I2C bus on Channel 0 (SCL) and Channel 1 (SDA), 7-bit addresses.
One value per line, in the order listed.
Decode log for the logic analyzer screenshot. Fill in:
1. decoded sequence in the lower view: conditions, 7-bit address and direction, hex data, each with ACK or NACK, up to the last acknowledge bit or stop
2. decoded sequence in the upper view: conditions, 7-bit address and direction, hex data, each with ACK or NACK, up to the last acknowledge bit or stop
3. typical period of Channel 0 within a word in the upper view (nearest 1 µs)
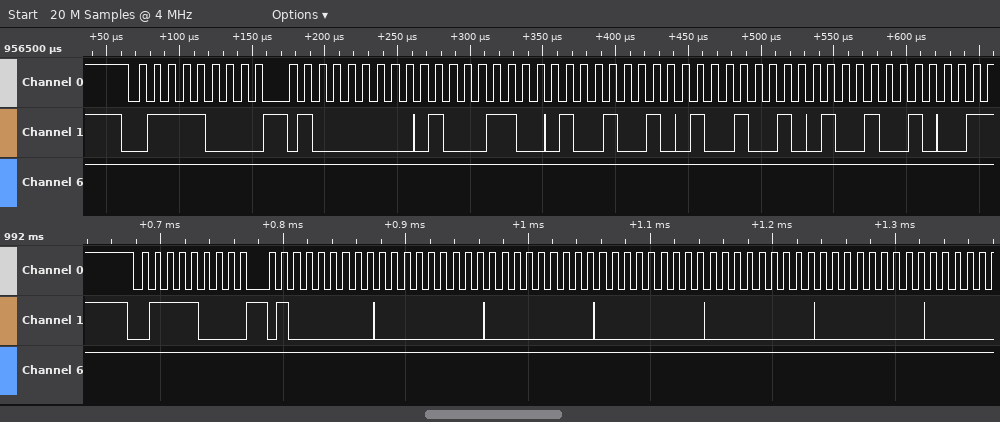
start, address 3C write ACK, 40 ACK, 00 ACK, 00 ACK, 00 ACK, 00 ACK, 00 ACK
start, address 3C write ACK, 40 ACK, 46 ACK, 49 ACK, 49 ACK, 49 ACK
10 µs
